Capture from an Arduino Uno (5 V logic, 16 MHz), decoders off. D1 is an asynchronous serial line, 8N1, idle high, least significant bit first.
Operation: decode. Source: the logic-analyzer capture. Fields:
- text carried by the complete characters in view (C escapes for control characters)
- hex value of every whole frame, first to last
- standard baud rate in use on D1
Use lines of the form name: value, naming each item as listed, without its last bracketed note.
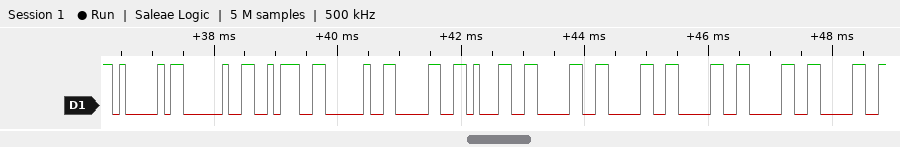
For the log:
text carried by the complete characters in view: "A : 0100000"
hex value of every whole frame, first to last: 41 20 3A 20 30 31 30 30 30 30 30
standard baud rate in use on D1: 9600 baud
